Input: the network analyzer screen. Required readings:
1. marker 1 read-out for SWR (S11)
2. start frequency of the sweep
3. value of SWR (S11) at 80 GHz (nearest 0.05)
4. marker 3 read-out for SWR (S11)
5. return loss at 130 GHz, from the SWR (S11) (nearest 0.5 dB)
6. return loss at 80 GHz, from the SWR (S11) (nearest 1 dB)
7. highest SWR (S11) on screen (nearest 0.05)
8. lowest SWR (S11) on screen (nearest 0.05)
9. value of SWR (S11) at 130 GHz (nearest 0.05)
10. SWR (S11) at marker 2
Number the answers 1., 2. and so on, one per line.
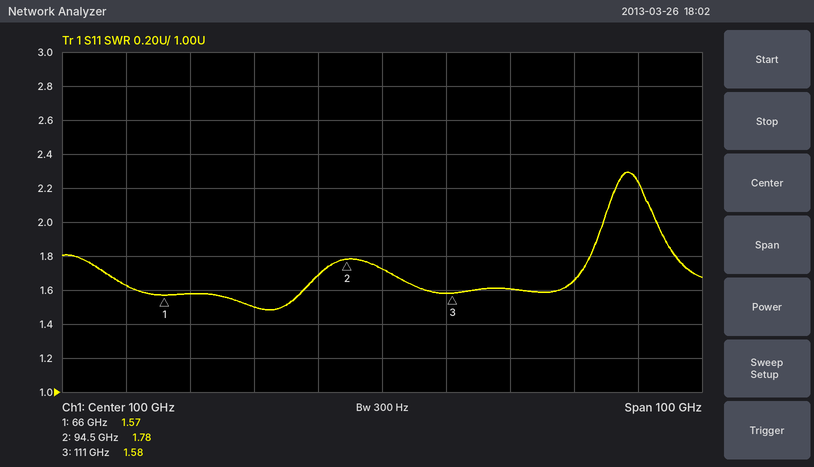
1. 1.57
2. 50 GHz
3. 1.50
4. 1.58
5. 12.0 dB
6. 14 dB
7. 2.30
8. 1.50
9. 1.65
10. 1.78
